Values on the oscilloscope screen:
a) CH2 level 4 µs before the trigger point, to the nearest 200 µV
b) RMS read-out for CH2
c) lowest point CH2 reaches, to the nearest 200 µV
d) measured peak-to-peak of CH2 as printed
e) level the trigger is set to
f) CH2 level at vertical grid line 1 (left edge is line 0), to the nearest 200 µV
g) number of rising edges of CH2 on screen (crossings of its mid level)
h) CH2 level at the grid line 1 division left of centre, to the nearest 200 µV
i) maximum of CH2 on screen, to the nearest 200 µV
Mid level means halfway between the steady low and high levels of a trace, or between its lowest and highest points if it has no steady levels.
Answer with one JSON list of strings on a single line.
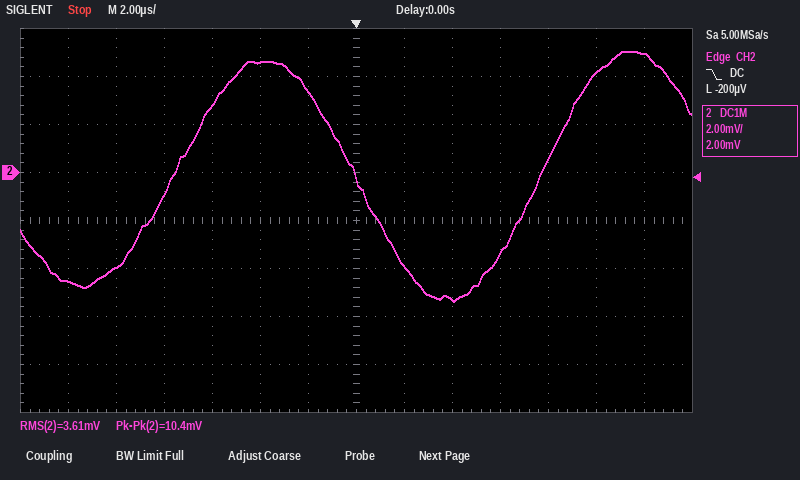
["4.6 mV", "3.61 mV", "-5.4 mV", "10.4 mV", "-200 µV", "-4.6 mV", "2", "3.4 mV", "5.0 mV"]
